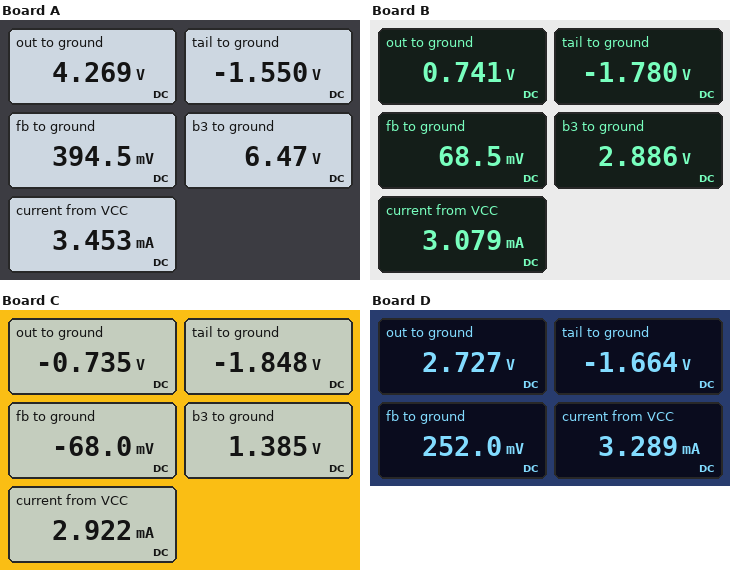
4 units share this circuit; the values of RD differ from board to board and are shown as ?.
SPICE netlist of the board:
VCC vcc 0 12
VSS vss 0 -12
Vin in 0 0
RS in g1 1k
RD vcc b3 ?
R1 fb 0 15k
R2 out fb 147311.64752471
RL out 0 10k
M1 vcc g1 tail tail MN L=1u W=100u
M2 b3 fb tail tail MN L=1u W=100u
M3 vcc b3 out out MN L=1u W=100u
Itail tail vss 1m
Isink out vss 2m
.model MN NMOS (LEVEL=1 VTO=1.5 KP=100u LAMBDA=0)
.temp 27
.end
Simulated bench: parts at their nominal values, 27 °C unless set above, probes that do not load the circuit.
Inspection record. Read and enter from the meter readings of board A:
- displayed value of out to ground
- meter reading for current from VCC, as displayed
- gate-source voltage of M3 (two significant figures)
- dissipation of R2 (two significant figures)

4.269 V
3.453 mA
2.2 V
100 µW
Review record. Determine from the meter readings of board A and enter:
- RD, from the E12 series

5.6 kΩ
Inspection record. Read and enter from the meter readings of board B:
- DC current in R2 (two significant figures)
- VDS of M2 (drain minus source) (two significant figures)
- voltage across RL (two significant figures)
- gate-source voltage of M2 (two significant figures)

4.6 µA
4.7 V
740 mV
1.8 V
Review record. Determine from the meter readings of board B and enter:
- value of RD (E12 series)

15 kΩ
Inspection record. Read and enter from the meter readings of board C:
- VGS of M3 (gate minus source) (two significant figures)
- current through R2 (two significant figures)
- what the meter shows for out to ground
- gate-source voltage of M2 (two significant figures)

2.1 V
4.5 µA
-0.735 V
1.8 V
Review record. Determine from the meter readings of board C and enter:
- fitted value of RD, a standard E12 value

27 kΩ
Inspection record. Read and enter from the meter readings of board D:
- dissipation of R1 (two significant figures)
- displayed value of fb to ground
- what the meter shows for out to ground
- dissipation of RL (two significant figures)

4.2 µW
252.0 mV
2.727 V
740 µW
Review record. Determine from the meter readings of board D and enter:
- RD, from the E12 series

8.2 kΩ
